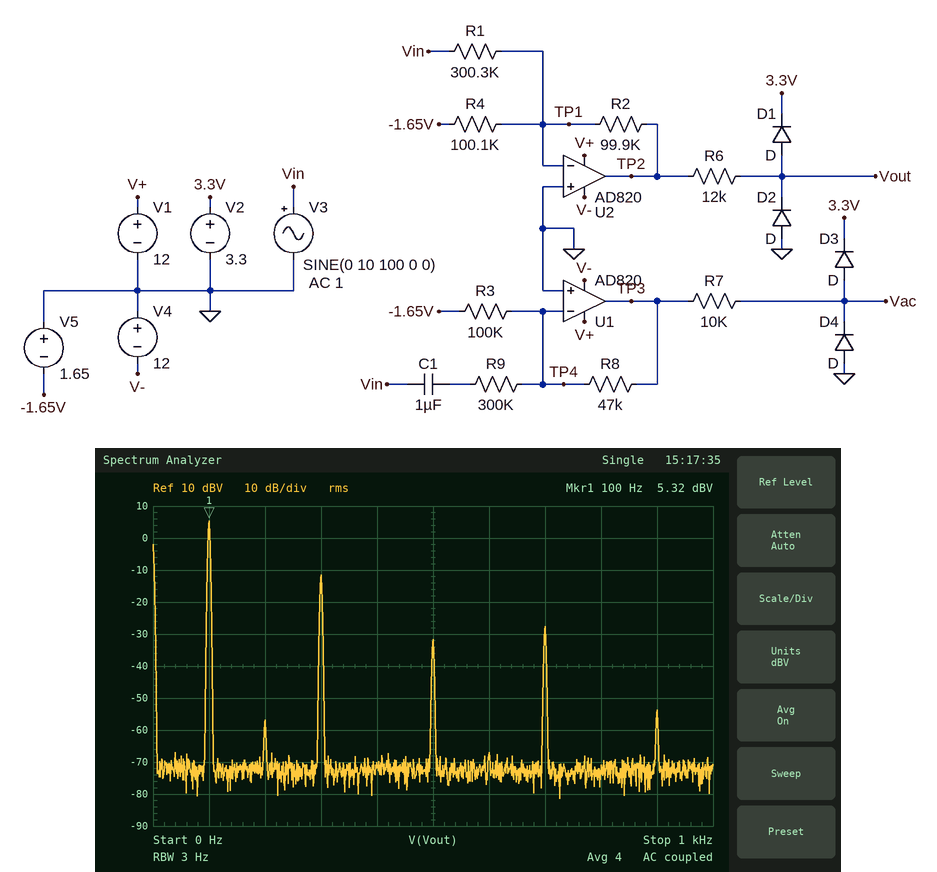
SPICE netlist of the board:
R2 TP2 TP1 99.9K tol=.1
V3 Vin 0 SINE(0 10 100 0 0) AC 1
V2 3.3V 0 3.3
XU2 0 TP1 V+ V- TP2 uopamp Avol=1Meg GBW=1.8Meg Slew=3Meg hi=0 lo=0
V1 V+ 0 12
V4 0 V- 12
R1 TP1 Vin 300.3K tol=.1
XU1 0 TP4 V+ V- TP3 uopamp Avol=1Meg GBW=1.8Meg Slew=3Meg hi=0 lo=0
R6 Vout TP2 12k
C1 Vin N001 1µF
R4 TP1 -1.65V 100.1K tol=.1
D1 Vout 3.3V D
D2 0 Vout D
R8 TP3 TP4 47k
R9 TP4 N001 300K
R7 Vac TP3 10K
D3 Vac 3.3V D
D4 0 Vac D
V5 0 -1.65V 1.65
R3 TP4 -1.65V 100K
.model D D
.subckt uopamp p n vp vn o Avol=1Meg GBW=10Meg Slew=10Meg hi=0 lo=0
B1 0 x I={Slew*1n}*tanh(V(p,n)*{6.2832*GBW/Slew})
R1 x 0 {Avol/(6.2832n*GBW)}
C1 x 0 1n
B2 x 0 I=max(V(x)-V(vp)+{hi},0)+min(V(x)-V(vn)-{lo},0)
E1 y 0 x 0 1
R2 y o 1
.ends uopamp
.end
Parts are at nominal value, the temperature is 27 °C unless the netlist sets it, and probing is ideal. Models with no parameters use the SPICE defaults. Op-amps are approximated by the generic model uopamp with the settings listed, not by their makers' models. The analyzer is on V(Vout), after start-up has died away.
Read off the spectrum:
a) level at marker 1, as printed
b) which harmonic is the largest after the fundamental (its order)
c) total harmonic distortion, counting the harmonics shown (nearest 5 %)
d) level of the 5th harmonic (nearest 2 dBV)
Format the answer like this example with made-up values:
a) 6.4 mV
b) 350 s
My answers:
a) 5.32 dBV
b) 3
c) 15 %
d) -32 dBV
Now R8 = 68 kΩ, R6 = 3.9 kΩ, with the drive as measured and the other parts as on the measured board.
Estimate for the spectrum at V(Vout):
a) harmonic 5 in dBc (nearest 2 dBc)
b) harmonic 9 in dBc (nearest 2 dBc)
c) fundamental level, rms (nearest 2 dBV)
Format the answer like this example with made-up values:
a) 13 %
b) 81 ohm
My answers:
a) -36 dBc
b) -52 dBc
c) 6 dBV
